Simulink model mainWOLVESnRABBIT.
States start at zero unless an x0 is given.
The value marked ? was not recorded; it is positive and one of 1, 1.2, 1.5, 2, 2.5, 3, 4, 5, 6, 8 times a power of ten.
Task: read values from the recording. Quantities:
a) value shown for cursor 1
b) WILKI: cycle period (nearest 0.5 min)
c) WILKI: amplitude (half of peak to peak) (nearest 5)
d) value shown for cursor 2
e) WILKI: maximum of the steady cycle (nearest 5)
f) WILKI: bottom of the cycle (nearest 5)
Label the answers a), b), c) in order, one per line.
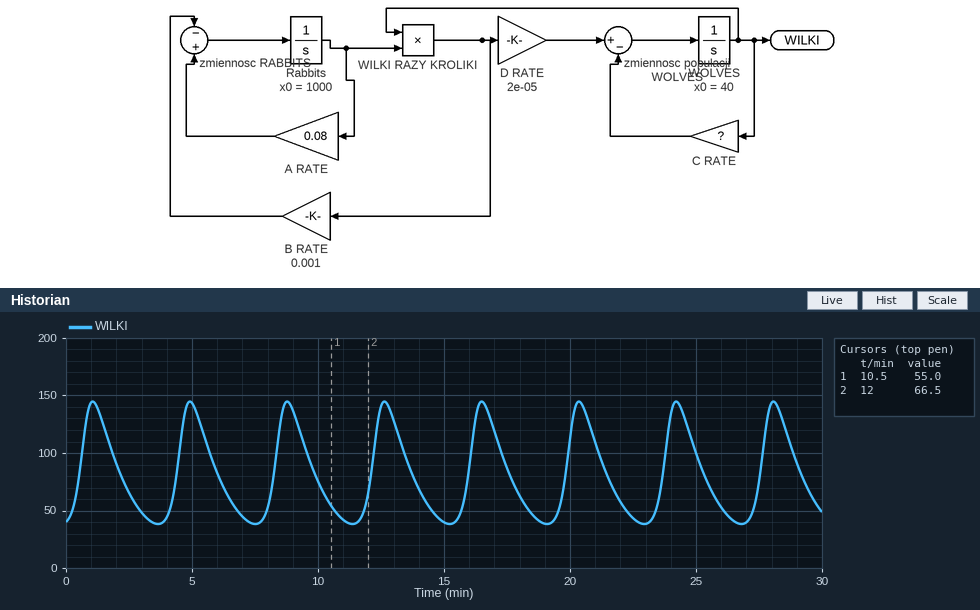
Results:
a) 55.0
b) 4.0 min
c) 55
d) 66.5
e) 145
f) 40
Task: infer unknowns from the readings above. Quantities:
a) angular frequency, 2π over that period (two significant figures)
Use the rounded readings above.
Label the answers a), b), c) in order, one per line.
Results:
a) 1.6 rad/min
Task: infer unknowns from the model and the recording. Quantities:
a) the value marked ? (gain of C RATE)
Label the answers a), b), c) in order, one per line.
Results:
a) 0.012
